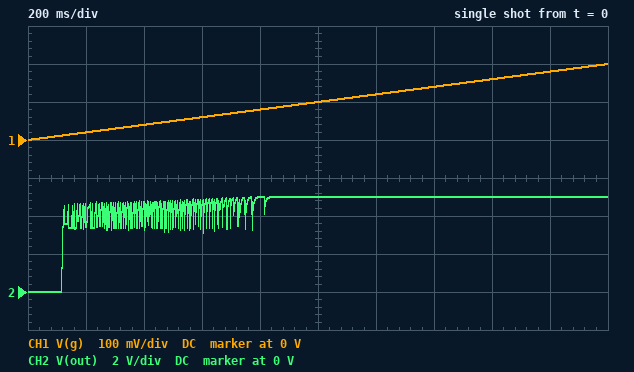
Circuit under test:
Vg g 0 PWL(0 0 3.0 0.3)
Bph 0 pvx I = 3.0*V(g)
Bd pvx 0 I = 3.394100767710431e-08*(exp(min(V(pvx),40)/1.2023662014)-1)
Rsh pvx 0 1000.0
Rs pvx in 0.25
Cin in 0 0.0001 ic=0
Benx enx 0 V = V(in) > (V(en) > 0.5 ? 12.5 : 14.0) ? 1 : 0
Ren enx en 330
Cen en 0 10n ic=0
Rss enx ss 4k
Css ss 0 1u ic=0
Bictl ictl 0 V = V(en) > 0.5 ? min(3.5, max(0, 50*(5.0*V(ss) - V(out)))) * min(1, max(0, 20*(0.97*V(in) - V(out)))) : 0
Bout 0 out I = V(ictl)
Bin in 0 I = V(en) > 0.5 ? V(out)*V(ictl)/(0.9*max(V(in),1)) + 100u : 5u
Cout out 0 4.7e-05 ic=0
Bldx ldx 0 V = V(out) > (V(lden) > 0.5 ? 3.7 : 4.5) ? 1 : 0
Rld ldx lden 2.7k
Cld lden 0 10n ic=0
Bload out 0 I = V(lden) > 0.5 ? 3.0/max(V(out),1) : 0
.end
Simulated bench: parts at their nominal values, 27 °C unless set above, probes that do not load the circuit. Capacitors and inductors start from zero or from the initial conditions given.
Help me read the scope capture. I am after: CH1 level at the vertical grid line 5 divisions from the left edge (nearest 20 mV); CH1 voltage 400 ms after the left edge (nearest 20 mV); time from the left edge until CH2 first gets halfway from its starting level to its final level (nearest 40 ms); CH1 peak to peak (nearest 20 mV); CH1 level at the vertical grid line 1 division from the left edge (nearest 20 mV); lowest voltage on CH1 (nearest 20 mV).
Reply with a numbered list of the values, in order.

1. 100 mV
2. 40 mV
3. 120 ms
4. 200 mV
5. 20 mV
6. 0 V
